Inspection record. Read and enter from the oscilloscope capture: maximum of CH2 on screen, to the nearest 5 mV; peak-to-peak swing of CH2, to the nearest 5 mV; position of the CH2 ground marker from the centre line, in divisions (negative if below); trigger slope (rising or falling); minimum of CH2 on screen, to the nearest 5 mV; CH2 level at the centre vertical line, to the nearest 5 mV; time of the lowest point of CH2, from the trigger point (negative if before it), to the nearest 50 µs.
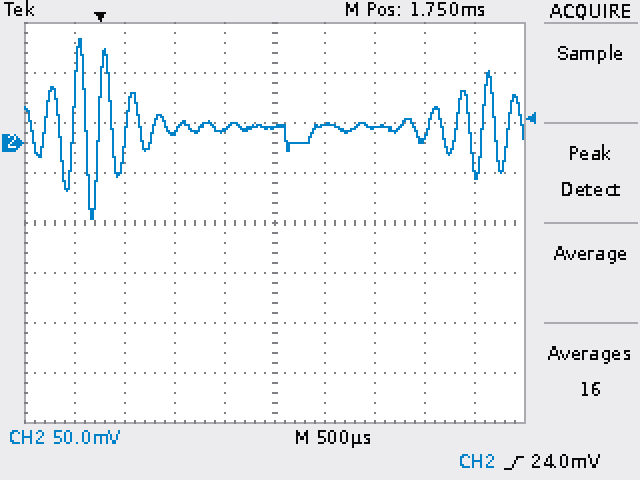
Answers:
105 mV
180 mV
+1.6 div
rising
-75 mV
15 mV
-50 µs
